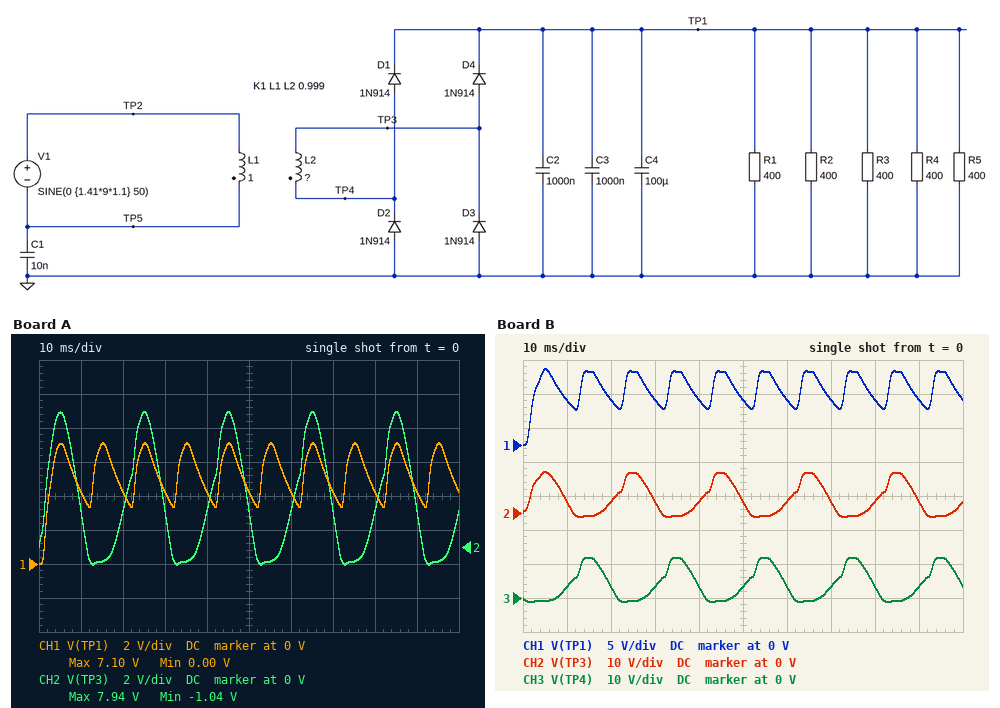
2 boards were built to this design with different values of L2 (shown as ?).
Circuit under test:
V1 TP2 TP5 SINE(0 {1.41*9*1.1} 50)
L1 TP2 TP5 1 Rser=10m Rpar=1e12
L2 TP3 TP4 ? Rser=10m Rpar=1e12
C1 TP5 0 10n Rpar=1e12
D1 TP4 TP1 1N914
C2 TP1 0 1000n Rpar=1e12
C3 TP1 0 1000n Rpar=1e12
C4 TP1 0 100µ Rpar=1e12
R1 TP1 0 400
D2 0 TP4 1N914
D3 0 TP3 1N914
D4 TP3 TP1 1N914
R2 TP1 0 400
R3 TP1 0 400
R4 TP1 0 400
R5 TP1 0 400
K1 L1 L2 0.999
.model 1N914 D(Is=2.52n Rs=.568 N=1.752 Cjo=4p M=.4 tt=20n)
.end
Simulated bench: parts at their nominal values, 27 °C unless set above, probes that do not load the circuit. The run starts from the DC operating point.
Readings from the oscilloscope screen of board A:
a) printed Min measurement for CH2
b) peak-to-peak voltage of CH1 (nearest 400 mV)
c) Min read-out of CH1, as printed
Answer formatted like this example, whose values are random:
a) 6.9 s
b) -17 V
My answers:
a) -1.04 V
b) 7.2 V
c) 0.00 V
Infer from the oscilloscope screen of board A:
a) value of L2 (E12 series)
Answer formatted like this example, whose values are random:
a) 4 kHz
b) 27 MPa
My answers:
a) 390 mH
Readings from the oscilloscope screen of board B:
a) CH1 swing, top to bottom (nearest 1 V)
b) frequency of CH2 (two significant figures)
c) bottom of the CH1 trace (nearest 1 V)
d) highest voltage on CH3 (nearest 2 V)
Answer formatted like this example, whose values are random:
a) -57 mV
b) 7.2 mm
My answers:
a) 11 V
b) 50 Hz
c) 0 V
d) 12 V
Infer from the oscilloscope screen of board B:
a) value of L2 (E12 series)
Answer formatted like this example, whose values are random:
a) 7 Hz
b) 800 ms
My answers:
a) 820 mH
